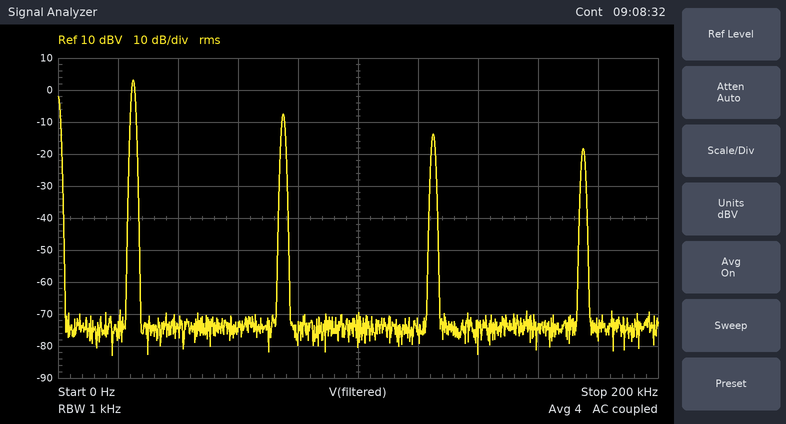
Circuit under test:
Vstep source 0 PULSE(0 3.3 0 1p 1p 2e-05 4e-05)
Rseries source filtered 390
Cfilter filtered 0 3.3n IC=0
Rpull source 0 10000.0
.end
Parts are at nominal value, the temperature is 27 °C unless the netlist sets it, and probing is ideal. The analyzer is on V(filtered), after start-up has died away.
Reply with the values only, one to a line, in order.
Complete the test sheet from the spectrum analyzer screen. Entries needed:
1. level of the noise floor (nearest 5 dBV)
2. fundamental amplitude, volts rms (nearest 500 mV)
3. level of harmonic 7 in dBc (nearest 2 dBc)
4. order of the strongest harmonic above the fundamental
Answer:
-75 dBV
1.5 V
-22 dBc
3
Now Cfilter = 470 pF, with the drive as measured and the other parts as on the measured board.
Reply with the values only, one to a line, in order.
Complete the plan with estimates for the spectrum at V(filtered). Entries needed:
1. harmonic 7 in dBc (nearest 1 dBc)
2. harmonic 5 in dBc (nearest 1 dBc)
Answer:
-17 dBc
-14 dBc
